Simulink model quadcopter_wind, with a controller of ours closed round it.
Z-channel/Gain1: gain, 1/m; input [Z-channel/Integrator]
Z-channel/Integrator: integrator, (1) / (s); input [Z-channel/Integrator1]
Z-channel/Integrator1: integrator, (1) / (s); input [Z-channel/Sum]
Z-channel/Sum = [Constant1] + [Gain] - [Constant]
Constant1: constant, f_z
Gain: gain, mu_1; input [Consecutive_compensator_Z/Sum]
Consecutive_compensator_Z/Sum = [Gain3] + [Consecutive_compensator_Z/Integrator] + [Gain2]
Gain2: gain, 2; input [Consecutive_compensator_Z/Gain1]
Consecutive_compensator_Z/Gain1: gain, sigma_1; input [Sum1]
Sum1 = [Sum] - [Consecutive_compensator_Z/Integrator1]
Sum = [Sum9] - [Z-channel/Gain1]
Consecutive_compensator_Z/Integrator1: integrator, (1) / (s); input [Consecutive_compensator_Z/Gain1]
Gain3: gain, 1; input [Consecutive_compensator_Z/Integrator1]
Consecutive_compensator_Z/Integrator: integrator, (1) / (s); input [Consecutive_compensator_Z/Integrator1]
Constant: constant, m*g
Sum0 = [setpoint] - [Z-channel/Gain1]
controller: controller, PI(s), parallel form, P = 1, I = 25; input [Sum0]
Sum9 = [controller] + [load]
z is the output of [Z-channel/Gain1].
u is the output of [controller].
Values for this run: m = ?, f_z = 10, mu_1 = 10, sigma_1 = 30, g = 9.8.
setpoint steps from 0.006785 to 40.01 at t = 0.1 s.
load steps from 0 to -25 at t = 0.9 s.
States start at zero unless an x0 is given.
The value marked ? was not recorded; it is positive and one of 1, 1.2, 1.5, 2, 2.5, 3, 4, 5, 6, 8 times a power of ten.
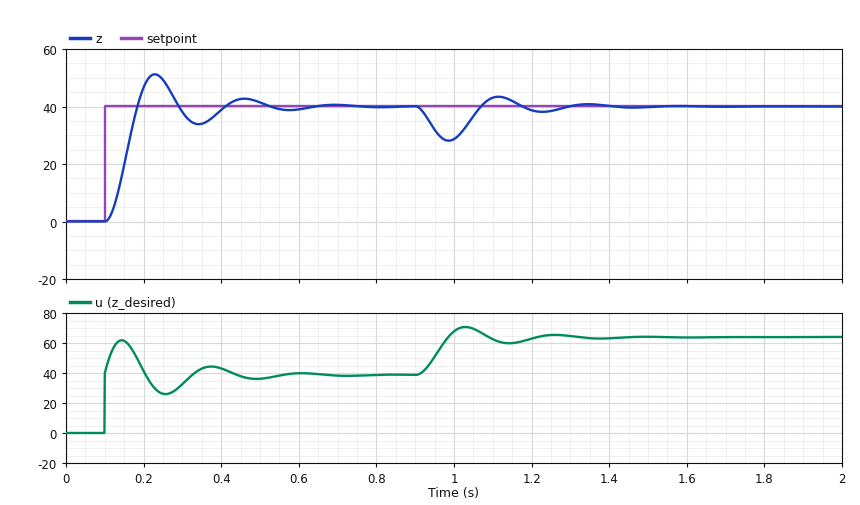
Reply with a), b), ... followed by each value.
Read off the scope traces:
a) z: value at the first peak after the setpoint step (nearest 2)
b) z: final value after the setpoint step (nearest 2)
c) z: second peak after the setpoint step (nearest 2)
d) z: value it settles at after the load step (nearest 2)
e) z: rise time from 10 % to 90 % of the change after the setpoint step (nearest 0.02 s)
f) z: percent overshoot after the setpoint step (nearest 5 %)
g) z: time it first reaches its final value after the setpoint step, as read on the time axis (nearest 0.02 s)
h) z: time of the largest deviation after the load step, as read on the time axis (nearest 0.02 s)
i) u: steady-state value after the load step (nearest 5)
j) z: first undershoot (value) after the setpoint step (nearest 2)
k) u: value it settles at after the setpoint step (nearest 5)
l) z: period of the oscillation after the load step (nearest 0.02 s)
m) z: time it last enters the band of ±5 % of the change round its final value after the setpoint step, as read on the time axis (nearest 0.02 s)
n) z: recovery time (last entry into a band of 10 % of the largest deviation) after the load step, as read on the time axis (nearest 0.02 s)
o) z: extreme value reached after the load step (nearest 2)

a) 52
b) 40
c) 42
d) 40
e) 0.06 s
f) 30 %
g) 0.18 s
h) 0.98 s
i) 65
j) 34
k) 40
l) 0.24 s
m) 0.48 s
n) 1.26 s
o) 28
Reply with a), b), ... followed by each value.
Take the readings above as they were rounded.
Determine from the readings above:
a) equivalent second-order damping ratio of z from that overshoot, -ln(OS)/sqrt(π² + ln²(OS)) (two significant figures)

a) 0.36
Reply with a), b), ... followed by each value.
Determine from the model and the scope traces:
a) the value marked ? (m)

a) 1.2
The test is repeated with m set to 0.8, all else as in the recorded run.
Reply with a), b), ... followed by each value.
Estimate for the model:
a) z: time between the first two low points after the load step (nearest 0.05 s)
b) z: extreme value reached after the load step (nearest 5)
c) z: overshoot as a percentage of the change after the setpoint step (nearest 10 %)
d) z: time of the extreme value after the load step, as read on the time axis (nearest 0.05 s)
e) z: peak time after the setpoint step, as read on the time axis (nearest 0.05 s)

a) 0.20 s
b) 25
c) 20 %
d) 0.95 s
e) 0.20 s
